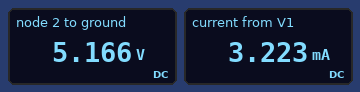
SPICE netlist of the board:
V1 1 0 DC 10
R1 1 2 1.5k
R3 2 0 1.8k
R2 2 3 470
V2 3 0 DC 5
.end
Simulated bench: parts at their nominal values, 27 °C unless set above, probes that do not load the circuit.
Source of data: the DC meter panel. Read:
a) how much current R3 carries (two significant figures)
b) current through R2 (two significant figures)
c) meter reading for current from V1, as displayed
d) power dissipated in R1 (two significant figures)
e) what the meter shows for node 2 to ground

2.9 mA
350 µA
3.223 mA
16 mW
5.166 V
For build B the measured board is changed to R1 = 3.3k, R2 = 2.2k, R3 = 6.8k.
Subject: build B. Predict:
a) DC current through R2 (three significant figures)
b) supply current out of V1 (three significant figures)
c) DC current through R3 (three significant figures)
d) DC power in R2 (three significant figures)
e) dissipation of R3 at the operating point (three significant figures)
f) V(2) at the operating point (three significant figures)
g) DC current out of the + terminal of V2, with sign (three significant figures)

392 µA
1.25 mA
862 µA
338 µW
5.05 mW
5.86 V
-392 µA
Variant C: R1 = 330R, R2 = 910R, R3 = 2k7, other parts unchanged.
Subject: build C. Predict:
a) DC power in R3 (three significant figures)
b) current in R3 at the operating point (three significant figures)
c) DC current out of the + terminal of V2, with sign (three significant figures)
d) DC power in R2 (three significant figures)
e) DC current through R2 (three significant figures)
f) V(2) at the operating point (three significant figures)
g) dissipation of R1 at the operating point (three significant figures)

23.4 mW
2.95 mA
-3.25 mA
9.60 mW
3.25 mA
7.96 V
12.7 mW
